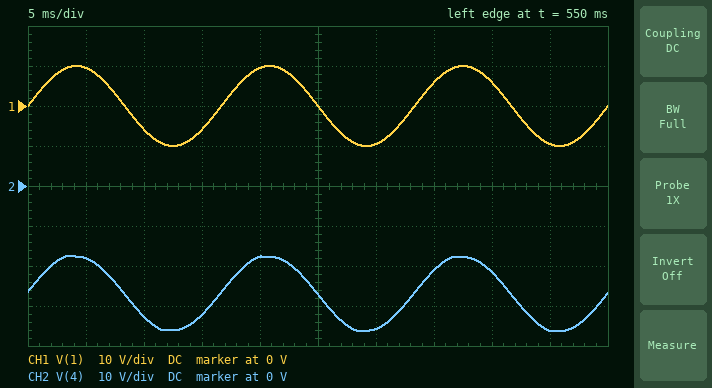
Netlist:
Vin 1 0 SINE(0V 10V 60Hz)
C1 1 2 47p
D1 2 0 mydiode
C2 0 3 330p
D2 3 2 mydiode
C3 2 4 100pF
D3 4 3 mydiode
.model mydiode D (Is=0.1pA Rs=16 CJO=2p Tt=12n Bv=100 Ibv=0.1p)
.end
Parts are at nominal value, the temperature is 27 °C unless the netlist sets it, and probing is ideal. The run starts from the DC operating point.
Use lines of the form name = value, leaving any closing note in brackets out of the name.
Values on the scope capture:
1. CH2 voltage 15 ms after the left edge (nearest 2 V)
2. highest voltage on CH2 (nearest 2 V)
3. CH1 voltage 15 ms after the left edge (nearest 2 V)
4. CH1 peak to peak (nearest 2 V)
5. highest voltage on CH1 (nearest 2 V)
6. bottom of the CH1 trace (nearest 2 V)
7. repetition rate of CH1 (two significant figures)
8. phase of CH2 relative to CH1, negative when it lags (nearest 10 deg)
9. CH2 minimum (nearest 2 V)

CH2 voltage 15 ms after the left edge = -32 V
highest voltage on CH2 = -18 V
CH1 voltage 15 ms after the left edge = -6 V
CH1 peak to peak = 20 V
highest voltage on CH1 = 10 V
bottom of the CH1 trace = -10 V
repetition rate of CH1 = 60 Hz
phase of CH2 relative to CH1, negative when it lags = 0 deg
CH2 minimum = -36 V
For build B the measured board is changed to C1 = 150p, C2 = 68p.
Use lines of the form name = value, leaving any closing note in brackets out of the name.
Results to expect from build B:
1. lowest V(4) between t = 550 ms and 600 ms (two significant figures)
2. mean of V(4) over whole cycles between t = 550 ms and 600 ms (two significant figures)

lowest V(4) between t = 550 ms and 600 ms = -38 V
mean of V(4) over whole cycles between t = 550 ms and 600 ms = -28 V
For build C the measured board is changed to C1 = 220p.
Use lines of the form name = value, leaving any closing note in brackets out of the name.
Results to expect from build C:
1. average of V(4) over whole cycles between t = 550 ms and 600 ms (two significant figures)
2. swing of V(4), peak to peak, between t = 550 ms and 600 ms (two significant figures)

average of V(4) over whole cycles between t = 550 ms and 600 ms = -29 V
swing of V(4), peak to peak, between t = 550 ms and 600 ms = 20 V
